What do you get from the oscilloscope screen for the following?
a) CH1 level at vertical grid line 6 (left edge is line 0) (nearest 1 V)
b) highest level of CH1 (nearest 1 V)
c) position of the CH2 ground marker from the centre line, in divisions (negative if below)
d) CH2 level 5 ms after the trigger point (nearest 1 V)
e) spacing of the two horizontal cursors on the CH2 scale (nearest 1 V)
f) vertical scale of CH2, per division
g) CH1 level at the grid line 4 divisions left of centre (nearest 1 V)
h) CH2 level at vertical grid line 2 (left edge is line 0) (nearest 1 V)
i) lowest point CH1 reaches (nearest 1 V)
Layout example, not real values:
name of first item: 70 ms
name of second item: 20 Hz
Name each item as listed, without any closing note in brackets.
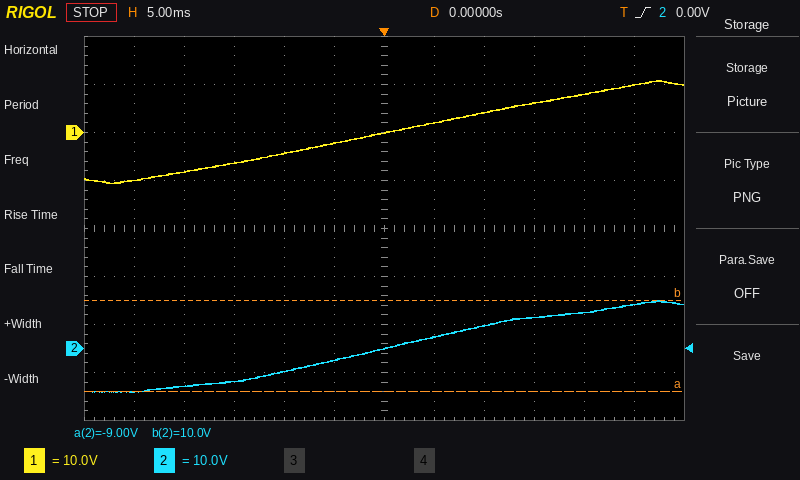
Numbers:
CH1 level at vertical grid line 6 (left edge is line 0): 0 V
highest level of CH1: 11 V
position of the CH2 ground marker from the centre line, in divisions: -2.5 div
CH2 level 5 ms after the trigger point: 2 V
spacing of the two horizontal cursors on the CH2 scale: 19 V
vertical scale of CH2, per division: 10 V
CH1 level at the grid line 4 divisions left of centre: -8 V
CH2 level at vertical grid line 2 (left edge is line 0): -8 V
lowest point CH1 reaches: -11 V
